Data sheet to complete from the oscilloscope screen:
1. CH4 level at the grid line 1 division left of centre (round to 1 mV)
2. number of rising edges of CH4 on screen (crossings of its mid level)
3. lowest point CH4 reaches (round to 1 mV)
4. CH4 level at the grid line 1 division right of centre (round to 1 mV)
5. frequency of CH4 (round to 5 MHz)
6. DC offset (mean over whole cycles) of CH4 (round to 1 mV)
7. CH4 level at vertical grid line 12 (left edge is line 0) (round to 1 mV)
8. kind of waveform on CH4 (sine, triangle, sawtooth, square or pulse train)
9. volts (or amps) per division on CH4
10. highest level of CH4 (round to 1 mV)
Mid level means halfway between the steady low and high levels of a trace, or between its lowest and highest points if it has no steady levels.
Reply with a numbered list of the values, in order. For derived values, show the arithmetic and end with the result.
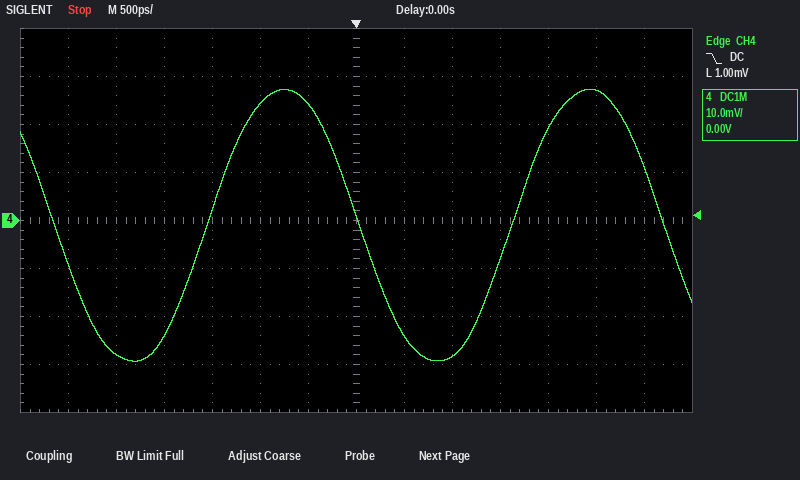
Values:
1. 24 mV
2. 2
3. -29 mV
4. -24 mV
5. 315 MHz
6. (27 mV + (-29 mV)) / 2 ≈ -1 mV
7. 27 mV
8. sine
9. 10 mV
10. 27 mV
